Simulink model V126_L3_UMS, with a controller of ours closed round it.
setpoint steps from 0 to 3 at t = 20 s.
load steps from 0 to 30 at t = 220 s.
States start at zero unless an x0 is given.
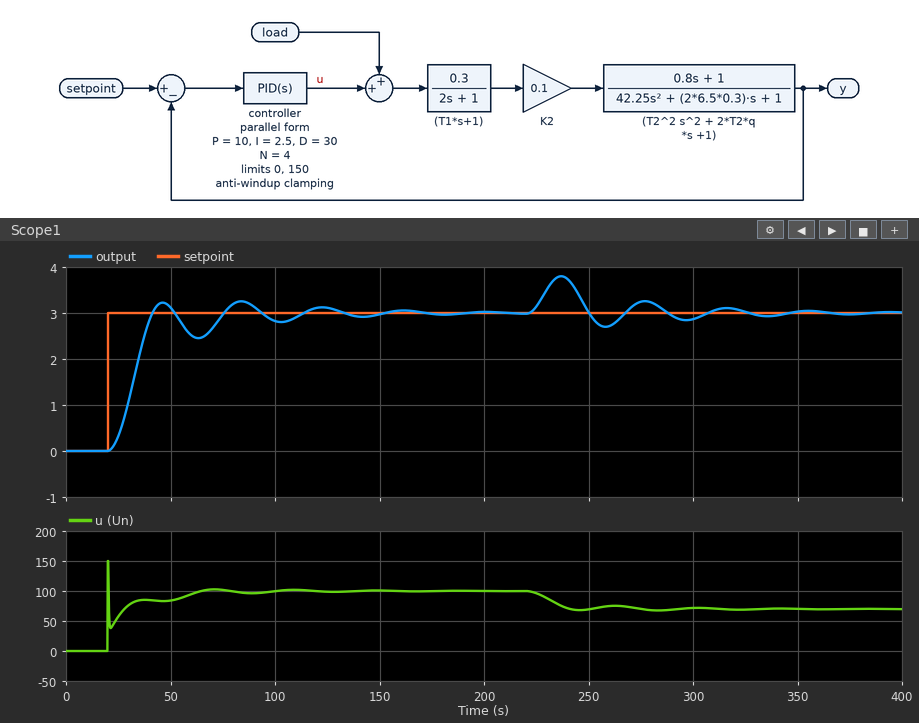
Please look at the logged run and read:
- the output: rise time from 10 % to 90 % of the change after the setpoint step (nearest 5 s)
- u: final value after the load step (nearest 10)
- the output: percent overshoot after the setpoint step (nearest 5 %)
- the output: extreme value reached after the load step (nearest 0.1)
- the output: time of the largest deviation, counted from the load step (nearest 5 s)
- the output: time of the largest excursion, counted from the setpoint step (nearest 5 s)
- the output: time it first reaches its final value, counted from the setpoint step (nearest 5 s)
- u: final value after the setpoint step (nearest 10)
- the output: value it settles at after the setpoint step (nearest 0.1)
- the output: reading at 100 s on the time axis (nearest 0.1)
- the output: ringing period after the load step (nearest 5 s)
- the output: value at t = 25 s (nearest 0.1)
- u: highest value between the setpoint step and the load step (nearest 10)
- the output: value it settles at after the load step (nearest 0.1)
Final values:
15 s
70
10 %
3.8
15 s
65 s
20 s
100
3.0
2.8
40 s
0.3
150
3.0
